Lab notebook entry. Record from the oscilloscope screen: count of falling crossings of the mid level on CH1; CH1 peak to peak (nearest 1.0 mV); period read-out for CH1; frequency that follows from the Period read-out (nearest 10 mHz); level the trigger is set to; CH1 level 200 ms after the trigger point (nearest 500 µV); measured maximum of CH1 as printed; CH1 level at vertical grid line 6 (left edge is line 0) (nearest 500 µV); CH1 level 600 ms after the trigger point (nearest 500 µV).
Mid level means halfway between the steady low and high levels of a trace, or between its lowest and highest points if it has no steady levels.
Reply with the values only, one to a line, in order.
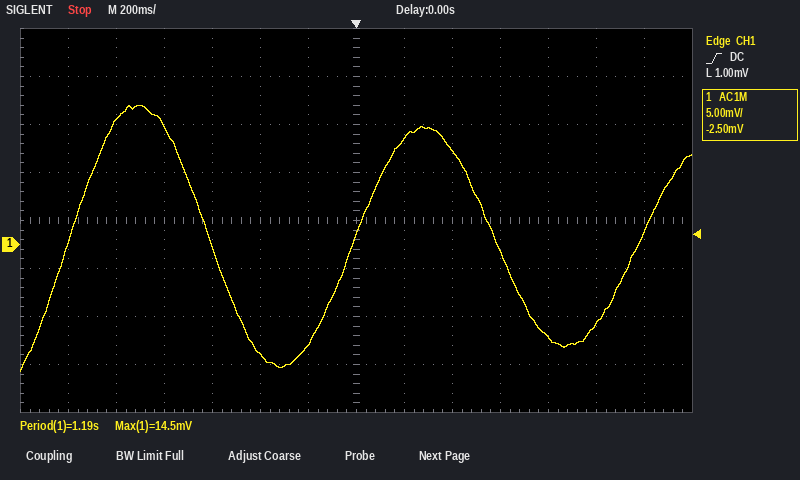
2
28.0 mV
1.19 s
840 mHz
1.00 mV
11.0 mV
14.5 mV
-10.5 mV
-500 µV
